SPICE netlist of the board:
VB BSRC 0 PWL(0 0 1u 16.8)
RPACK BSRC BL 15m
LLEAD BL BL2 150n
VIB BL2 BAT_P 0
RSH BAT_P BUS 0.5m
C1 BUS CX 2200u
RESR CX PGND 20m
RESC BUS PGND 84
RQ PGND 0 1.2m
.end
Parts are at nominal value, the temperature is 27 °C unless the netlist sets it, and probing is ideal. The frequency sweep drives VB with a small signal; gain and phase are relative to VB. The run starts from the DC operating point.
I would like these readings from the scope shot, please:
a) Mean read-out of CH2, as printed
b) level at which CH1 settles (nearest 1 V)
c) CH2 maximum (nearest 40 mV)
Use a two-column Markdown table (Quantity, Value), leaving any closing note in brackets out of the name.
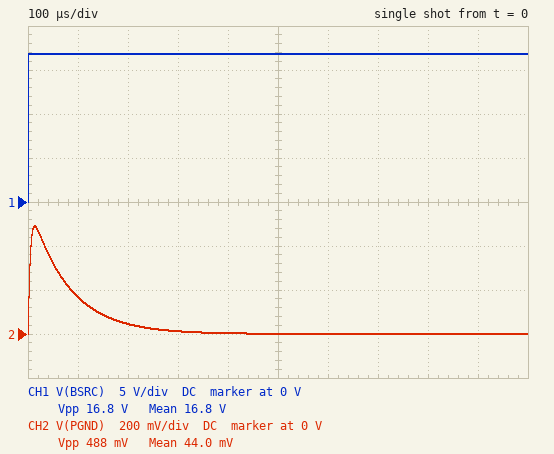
| Quantity | Value |
|---|---|
| Mean read-out of CH2, as printed | 44.0 mV |
| level at which CH1 settles | 17 V |
| CH2 maximum | 480 mV |
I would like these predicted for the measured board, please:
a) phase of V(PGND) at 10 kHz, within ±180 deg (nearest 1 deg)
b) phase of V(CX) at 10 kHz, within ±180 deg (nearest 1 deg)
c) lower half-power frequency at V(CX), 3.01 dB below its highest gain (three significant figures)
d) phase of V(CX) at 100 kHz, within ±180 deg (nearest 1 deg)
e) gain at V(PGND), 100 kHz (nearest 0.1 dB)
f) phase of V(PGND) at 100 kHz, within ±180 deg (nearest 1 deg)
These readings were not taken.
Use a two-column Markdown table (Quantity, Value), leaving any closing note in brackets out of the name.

| Quantity | Value |
|---|---|
| phase of V(PGND) at 10 kHz, within ±180 deg | -3 deg |
| phase of V(CX) at 10 kHz, within ±180 deg | -3 deg |
| lower half-power frequency at V(CX), 3.01 dB below its highest gain | 1.88 kHz |
| phase of V(CX) at 100 kHz, within ±180 deg | -69 deg |
| gain at V(PGND), 100 kHz | -38.5 dB |
| phase of V(PGND) at 100 kHz, within ±180 deg | -69 deg |
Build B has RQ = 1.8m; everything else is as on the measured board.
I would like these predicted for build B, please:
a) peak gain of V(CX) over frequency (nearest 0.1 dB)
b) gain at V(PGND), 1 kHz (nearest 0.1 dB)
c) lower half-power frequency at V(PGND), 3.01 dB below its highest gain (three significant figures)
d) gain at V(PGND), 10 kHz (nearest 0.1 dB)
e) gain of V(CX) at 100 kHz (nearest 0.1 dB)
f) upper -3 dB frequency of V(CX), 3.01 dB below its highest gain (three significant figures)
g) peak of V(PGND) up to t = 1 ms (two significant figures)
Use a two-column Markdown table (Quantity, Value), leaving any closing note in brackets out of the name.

| Quantity | Value |
|---|---|
| peak gain of V(CX) over frequency | -4.7 dB |
| gain at V(PGND), 1 kHz | -33.0 dB |
| lower half-power frequency at V(PGND), 3.01 dB below its highest gain | 1.85 kHz |
| gain at V(PGND), 10 kHz | -26.3 dB |
| gain of V(CX) at 100 kHz | -13.3 dB |
| upper -3 dB frequency of V(CX), 3.01 dB below its highest gain | 41.4 kHz |
| peak of V(PGND) up to t = 1 ms | 720 mV |
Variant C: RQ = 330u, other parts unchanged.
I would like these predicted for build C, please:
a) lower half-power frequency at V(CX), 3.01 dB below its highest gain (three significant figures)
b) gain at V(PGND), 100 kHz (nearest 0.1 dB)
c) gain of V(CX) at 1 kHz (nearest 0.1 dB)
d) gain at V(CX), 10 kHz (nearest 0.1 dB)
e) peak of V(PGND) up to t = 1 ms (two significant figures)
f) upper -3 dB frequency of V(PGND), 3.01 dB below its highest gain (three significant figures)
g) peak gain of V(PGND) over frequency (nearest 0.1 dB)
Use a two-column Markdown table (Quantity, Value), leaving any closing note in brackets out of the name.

| Quantity | Value |
|---|---|
| lower half-power frequency at V(CX), 3.01 dB below its highest gain | 1.92 kHz |
| gain at V(PGND), 100 kHz | -49.6 dB |
| gain of V(CX) at 1 kHz | -11.9 dB |
| gain at V(CX), 10 kHz | -4.9 dB |
| peak of V(PGND) up to t = 1 ms | 140 mV |
| upper -3 dB frequency of V(PGND), 3.01 dB below its highest gain | 39.9 kHz |
| peak gain of V(PGND) over frequency | -40.7 dB |
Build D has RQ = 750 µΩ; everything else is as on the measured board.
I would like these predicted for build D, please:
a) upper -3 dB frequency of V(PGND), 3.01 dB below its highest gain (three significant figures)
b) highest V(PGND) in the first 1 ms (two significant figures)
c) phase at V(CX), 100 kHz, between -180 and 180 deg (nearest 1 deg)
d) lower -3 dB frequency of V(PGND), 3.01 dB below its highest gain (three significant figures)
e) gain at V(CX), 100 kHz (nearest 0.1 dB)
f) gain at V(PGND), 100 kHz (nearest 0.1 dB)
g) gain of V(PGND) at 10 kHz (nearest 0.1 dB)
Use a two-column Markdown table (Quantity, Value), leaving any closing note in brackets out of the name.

| Quantity | Value |
|---|---|
| upper -3 dB frequency of V(PGND), 3.01 dB below its highest gain | 40.4 kHz |
| highest V(PGND) in the first 1 ms | 310 mV |
| phase at V(CX), 100 kHz, between -180 and 180 deg | -69 deg |
| lower -3 dB frequency of V(PGND), 3.01 dB below its highest gain | 1.90 kHz |
| gain at V(CX), 100 kHz | -13.7 dB |
| gain at V(PGND), 100 kHz | -42.5 dB |
| gain of V(PGND) at 10 kHz | -33.7 dB |
